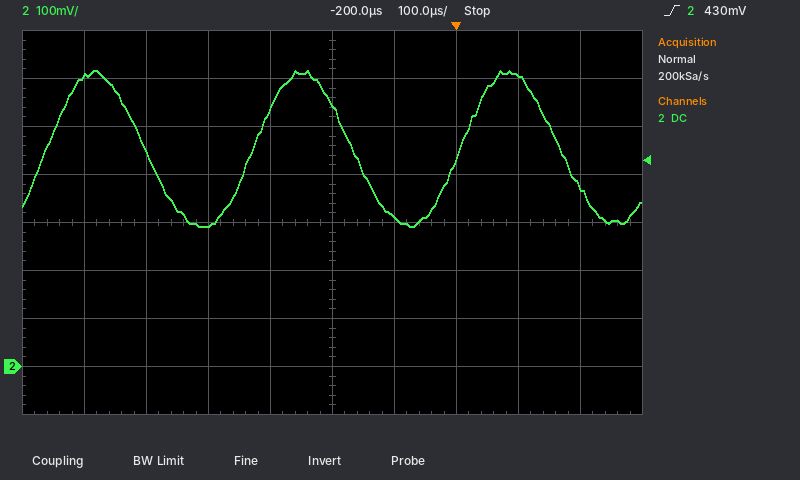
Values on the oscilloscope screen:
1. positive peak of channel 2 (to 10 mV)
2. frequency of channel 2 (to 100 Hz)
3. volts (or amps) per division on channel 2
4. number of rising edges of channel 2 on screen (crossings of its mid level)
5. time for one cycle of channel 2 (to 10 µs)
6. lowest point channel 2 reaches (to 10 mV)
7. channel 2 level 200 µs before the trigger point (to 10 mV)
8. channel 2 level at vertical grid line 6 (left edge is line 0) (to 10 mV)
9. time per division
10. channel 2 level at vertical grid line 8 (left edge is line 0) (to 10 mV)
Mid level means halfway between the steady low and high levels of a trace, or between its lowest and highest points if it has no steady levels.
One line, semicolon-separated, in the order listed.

620 mV; 3.0 kHz; 100 mV; 3; 330 µs; 290 mV; 550 mV; 310 mV; 100 µs; 610 mV
